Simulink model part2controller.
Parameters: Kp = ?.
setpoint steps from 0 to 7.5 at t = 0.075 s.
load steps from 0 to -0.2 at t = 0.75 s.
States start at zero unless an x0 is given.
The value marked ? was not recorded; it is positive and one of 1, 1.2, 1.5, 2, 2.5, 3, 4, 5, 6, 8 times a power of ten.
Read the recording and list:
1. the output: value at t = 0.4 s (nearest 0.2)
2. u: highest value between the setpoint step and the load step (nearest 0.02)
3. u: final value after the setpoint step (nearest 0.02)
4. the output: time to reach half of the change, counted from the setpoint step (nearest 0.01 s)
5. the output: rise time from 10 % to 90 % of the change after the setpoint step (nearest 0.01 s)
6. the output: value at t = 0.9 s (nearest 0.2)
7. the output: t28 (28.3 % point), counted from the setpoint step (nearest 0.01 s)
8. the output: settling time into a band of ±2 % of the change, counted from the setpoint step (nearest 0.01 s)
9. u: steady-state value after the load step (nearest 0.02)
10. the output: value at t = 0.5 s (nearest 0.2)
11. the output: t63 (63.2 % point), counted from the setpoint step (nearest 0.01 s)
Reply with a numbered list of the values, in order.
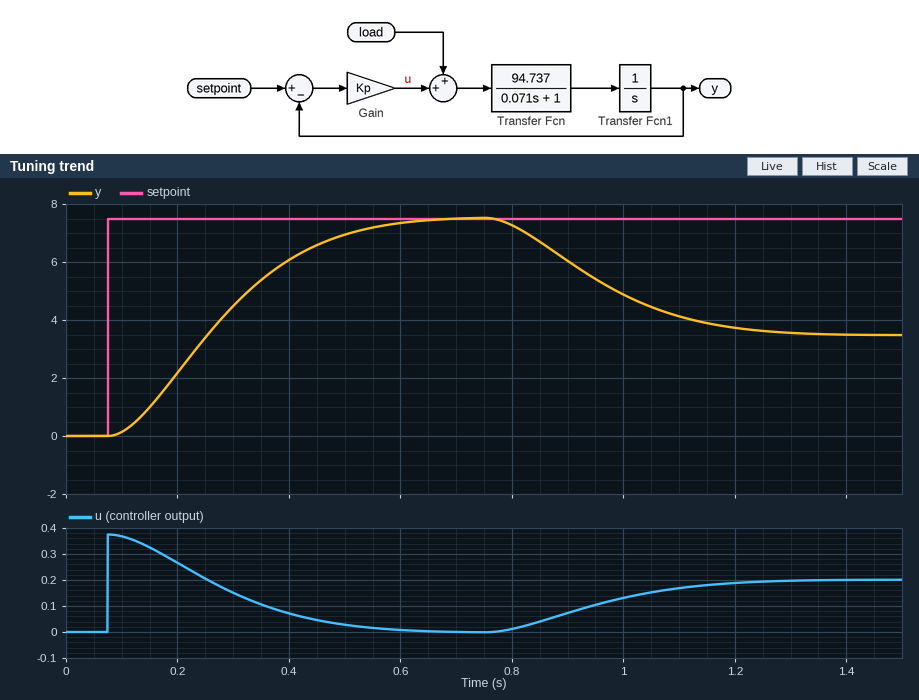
1. 6.0
2. 0.38
3. 0.00
4. 0.19 s
5. 0.33 s
6. 6.0
7. 0.12 s
8. 0.53 s
9. 0.20
10. 7.0
11. 0.24 s
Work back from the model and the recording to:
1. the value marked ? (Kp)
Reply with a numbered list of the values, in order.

1. 0.05
